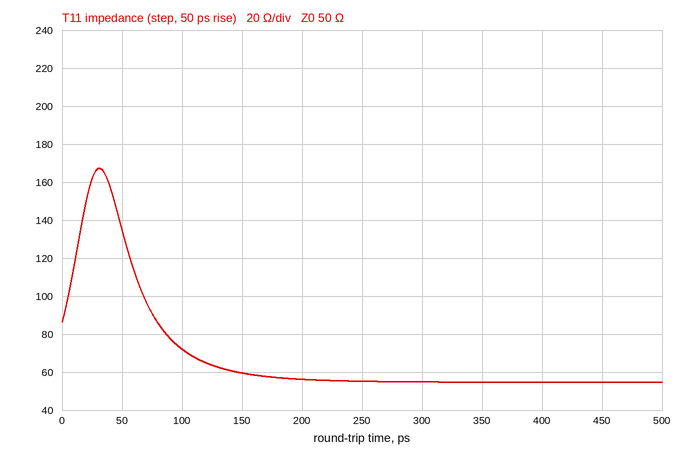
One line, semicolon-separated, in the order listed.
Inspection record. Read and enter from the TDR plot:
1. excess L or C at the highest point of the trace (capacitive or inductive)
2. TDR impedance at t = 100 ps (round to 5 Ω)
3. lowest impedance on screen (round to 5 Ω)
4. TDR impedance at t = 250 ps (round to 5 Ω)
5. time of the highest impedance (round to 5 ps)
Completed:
inductive; 70 Ω; 55 Ω; 55 Ω; 30 ps
